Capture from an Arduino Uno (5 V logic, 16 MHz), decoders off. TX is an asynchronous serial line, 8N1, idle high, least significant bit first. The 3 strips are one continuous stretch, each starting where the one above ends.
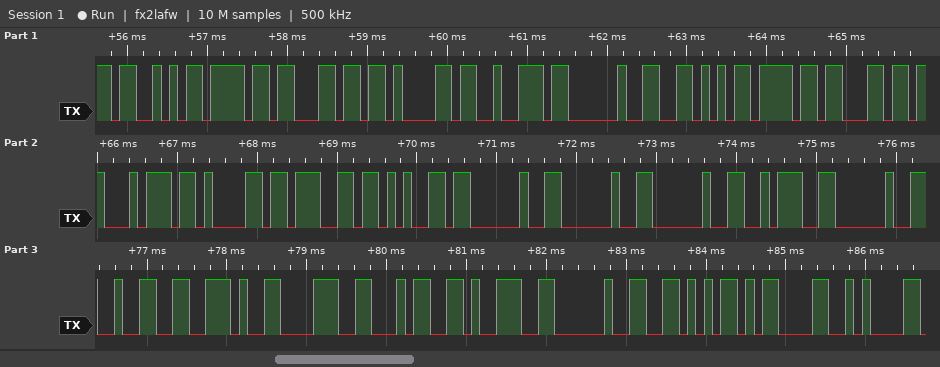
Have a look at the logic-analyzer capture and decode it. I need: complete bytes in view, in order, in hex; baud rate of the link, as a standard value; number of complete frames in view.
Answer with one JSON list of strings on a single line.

["53 6F 6C 61 72 20 56 6F 6C 74 61 67 65 20 20 20 3A 20 32 2E 38 34 39 20 56 0D 0A", "9600 baud", "27"]
